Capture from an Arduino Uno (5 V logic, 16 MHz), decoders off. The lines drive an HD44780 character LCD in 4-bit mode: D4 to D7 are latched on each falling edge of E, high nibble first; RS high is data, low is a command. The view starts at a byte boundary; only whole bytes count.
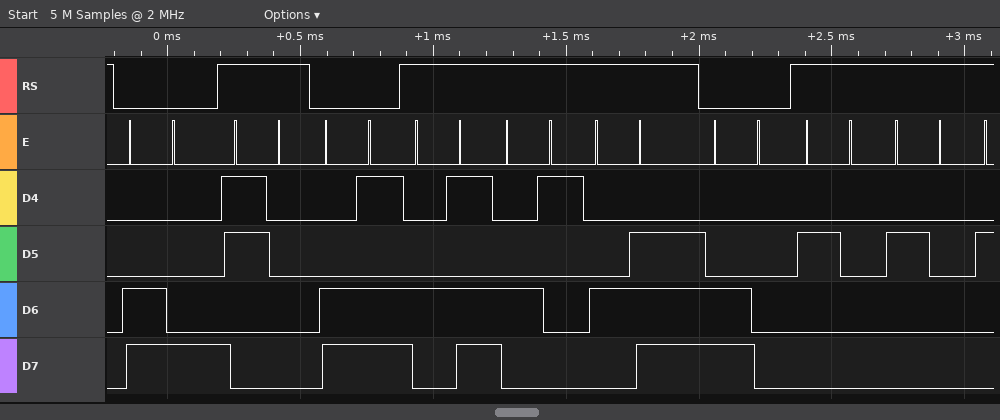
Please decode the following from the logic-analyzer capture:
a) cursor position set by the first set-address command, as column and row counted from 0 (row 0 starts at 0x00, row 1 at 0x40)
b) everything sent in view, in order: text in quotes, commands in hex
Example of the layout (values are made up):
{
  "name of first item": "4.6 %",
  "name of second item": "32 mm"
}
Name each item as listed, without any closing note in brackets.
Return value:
{
  "cursor position set by the first set-address command, as column and row counted from 0": "column 8, row 1",
  "everything sent in view, in order: text in quotes, commands in hex": "0xC8 \"0\" 0xCD \"MAN\" 0xC0 \"  \""
}
